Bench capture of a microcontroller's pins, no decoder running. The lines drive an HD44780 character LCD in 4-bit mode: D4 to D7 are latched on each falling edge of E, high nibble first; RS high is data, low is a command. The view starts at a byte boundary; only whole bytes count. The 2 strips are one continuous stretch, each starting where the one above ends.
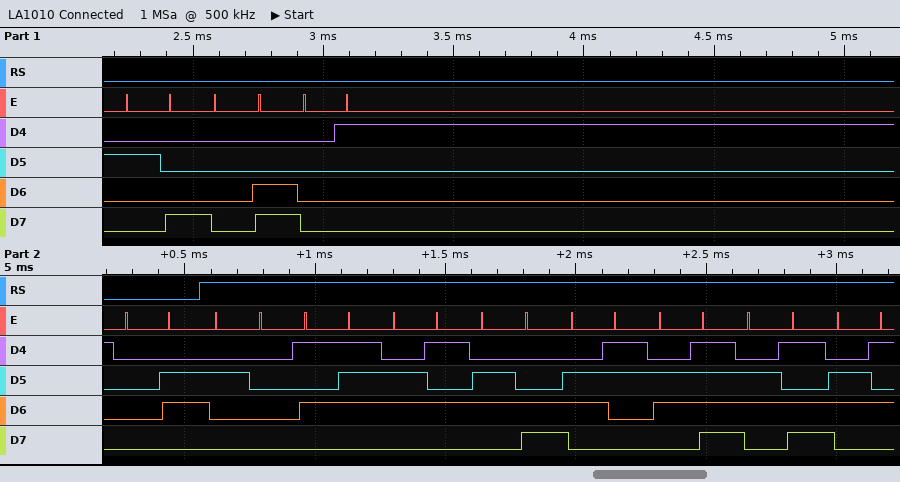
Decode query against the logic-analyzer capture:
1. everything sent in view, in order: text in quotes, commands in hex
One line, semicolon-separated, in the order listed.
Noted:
0x28 0x0C 0x01 0x06 " Welcome"
